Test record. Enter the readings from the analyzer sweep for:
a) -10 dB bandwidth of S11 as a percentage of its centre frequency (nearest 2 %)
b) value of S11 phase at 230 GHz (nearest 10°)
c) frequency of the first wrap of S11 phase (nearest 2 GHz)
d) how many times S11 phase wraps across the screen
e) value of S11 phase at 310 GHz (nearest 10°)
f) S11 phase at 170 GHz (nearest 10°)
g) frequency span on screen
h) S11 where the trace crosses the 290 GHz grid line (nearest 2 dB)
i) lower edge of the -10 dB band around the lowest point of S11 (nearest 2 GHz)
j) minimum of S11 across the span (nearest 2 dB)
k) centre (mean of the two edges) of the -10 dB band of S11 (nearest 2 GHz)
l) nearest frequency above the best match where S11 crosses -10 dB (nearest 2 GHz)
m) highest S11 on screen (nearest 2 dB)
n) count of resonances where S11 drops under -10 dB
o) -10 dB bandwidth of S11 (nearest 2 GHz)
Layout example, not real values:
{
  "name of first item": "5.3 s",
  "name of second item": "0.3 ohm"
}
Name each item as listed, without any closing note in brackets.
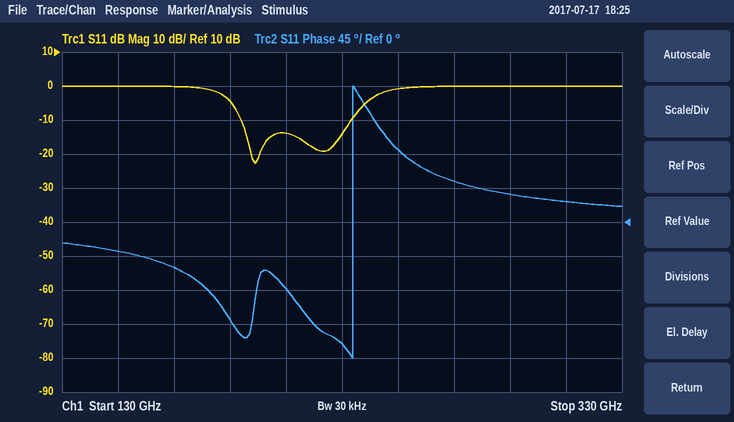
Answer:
{
  "-10 dB bandwidth of S11 as a percentage of its centre frequency": "18 %",
  "value of S11 phase at 230 GHz": "-160°",
  "frequency of the first wrap of S11 phase": "234 GHz",
  "how many times S11 phase wraps across the screen": "1",
  "value of S11 phase at 310 GHz": "30°",
  "S11 phase at 170 GHz": "-60°",
  "frequency span on screen": "200 GHz",
  "S11 where the trace crosses the 290 GHz grid line": "0 dB",
  "lower edge of the -10 dB band around the lowest point of S11": "194 GHz",
  "minimum of S11 across the span": "-22 dB",
  "centre (mean of the two edges) of the -10 dB band of S11": "214 GHz",
  "nearest frequency above the best match where S11 crosses -10 dB": "234 GHz",
  "highest S11 on screen": "0 dB",
  "count of resonances where S11 drops under -10 dB": "2",
  "-10 dB bandwidth of S11": "40 GHz"
}
